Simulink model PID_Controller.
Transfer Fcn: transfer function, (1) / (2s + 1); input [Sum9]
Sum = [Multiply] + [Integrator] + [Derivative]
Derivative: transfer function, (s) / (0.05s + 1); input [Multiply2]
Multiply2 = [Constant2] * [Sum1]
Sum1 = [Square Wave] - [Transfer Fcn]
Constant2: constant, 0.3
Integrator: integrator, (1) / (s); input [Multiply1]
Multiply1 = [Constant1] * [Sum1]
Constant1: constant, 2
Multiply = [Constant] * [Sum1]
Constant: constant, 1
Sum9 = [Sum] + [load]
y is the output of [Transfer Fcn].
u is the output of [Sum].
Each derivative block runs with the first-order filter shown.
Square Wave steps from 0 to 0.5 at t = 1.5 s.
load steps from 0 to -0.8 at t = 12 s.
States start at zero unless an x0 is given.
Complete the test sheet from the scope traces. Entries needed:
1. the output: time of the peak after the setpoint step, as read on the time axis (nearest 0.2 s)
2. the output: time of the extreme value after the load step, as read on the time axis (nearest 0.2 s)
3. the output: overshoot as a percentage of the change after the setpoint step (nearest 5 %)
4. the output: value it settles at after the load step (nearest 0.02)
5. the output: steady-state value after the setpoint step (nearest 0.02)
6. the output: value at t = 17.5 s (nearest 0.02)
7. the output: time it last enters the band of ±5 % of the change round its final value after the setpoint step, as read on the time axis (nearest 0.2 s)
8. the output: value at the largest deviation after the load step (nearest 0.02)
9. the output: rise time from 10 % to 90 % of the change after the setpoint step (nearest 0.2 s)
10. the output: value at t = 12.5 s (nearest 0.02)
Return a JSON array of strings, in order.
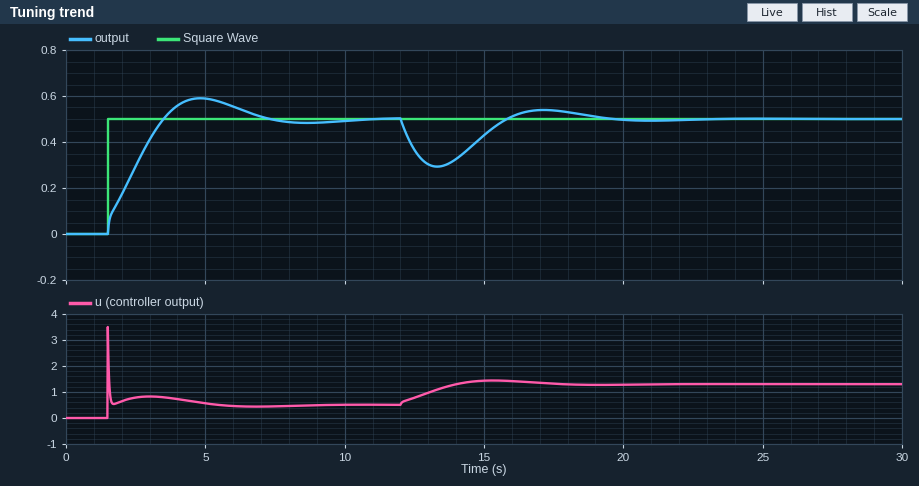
["4.8 s", "13.4 s", "20 %", "0.50", "0.50", "0.54", "6.6 s", "0.30", "1.6 s", "0.36"]
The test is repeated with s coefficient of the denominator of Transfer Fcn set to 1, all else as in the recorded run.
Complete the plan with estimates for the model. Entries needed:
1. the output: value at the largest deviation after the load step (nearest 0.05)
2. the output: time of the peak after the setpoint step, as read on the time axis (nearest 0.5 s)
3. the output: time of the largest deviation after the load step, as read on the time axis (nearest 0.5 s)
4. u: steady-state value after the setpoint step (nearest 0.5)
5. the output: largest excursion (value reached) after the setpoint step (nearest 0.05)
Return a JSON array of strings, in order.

["0.25", "4.5 s", "13.0 s", "0.5", "0.55"]
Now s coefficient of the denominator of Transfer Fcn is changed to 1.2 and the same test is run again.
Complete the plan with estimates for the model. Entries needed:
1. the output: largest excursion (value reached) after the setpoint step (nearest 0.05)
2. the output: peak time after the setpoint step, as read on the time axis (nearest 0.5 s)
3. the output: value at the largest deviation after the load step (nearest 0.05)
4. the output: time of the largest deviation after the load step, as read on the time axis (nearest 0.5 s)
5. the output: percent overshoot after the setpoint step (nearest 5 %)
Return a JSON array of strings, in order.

["0.55", "4.5 s", "0.25", "13.0 s", "10 %"]
